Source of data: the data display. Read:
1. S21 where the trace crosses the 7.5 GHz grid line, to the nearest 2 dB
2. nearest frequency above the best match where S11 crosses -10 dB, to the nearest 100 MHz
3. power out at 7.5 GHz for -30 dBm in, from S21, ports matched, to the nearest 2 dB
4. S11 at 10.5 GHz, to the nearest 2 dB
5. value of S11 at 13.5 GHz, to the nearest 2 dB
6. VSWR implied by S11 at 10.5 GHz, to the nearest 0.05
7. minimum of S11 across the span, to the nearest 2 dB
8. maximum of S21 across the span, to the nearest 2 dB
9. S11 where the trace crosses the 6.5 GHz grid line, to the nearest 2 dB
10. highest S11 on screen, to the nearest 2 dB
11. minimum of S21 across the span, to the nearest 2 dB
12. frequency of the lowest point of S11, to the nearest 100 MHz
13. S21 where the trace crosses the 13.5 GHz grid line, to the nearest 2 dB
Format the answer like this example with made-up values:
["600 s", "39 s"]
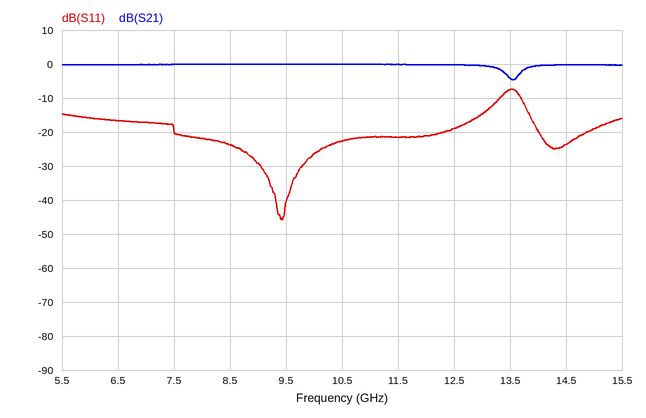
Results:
["0 dB", "13.3 GHz", "-30 dBm", "-22 dB", "-8 dB", "1.15", "-46 dB", "0 dB", "-16 dB", "-8 dB", "-4 dB", "9.4 GHz", "-4 dB"]
